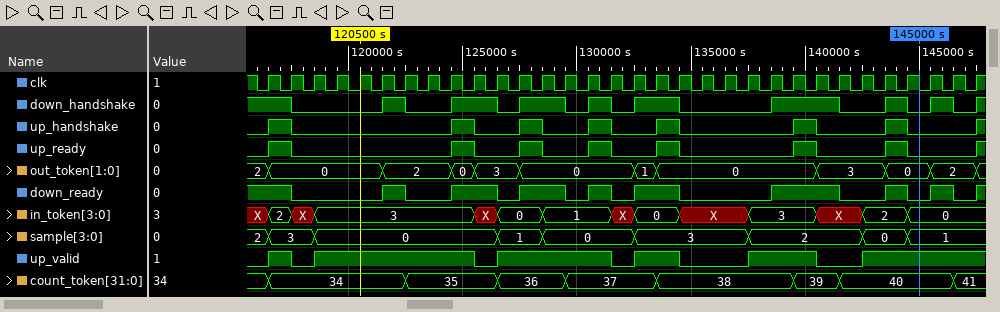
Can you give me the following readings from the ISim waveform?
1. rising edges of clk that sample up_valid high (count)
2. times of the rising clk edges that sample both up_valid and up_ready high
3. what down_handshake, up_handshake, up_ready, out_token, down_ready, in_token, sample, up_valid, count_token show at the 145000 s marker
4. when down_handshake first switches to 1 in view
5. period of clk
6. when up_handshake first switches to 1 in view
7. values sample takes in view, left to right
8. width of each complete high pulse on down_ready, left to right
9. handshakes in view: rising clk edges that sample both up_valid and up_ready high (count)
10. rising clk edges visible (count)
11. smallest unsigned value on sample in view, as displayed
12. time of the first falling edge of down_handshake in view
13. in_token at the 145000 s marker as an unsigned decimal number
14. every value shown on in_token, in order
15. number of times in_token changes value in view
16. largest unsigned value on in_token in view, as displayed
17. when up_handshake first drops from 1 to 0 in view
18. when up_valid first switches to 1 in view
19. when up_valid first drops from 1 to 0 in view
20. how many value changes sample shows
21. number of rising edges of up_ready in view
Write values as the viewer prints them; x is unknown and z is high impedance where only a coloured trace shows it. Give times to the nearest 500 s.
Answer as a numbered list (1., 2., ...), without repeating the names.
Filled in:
1. 23
2. 117500 s, 125500 s, 128500 s, 131500 s, 134500 s, 140500 s, 144500 s
3. down_handshake=0, up_handshake=0, up_ready=0, out_token=0, down_ready=0, in_token=0, sample=1, up_valid=1, count_token=40
4. 121500 s
5. 1000 s
6. 116500 s
7. 2, 3, 0, 1, 0, 3, 2, 0, 1
8. 1000 s, 2000 s, 2000 s, 1000 s, 2000 s, 3000 s, 1000 s, 1000 s
9. 7
10. 32
11. 0
12. 117500 s
13. 0
14. X, 2, X, 3, X, 0, 1, X, 0, X, 3, X, 2, 0
15. 13
16. 3
17. 117500 s
18. 116500 s
19. 117500 s
20. 8
21. 8
